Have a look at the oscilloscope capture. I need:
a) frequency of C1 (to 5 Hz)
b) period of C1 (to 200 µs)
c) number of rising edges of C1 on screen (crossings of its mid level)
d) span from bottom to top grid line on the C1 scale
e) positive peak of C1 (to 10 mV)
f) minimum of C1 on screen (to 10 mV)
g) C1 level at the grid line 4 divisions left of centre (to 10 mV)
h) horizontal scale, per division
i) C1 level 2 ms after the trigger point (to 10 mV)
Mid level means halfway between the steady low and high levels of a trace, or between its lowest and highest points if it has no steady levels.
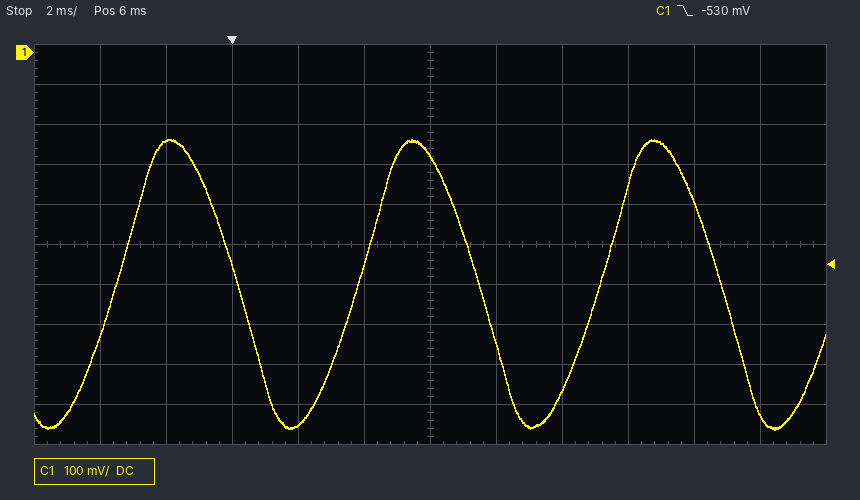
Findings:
135 Hz
7.4 ms
3
1 V
-220 mV
-940 mV
-220 mV
2 ms
-930 mV
